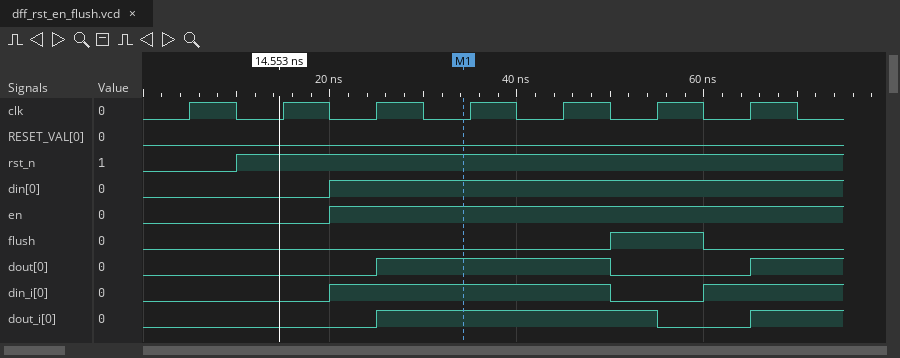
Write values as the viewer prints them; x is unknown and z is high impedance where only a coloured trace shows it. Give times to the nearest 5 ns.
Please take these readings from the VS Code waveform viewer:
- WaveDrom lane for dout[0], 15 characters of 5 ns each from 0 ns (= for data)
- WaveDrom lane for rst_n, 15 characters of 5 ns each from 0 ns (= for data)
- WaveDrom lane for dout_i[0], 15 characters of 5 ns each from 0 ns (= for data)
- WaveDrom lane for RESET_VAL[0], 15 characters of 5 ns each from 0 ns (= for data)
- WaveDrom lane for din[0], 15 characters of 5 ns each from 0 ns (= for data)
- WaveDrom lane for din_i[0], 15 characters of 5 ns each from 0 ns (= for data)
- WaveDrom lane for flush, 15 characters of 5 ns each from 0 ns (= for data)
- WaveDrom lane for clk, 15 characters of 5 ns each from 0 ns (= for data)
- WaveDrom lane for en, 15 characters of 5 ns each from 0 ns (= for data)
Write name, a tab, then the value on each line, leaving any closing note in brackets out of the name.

WaveDrom lane for dout[0], 15 characters of 5 ns each from 0 ns	{name: 'dout[0]', wave: '0....1....0..1.'}
WaveDrom lane for rst_n, 15 characters of 5 ns each from 0 ns	{name: 'rst_n', wave: '0.1............'}
WaveDrom lane for dout_i[0], 15 characters of 5 ns each from 0 ns	{name: 'dout_i[0]', wave: '0....1.....0.1.'}
WaveDrom lane for RESET_VAL[0], 15 characters of 5 ns each from 0 ns	{name: 'RESET_VAL[0]', wave: '0..............'}
WaveDrom lane for din[0], 15 characters of 5 ns each from 0 ns	{name: 'din[0]', wave: '0...1..........'}
WaveDrom lane for din_i[0], 15 characters of 5 ns each from 0 ns	{name: 'din_i[0]', wave: '0...1.....0.1..'}
WaveDrom lane for flush, 15 characters of 5 ns each from 0 ns	{name: 'flush', wave: '0.........1.0..'}
WaveDrom lane for clk, 15 characters of 5 ns each from 0 ns	{name: 'clk', wave: '010101010101010'}
WaveDrom lane for en, 15 characters of 5 ns each from 0 ns	{name: 'en', wave: '0...1..........'}
